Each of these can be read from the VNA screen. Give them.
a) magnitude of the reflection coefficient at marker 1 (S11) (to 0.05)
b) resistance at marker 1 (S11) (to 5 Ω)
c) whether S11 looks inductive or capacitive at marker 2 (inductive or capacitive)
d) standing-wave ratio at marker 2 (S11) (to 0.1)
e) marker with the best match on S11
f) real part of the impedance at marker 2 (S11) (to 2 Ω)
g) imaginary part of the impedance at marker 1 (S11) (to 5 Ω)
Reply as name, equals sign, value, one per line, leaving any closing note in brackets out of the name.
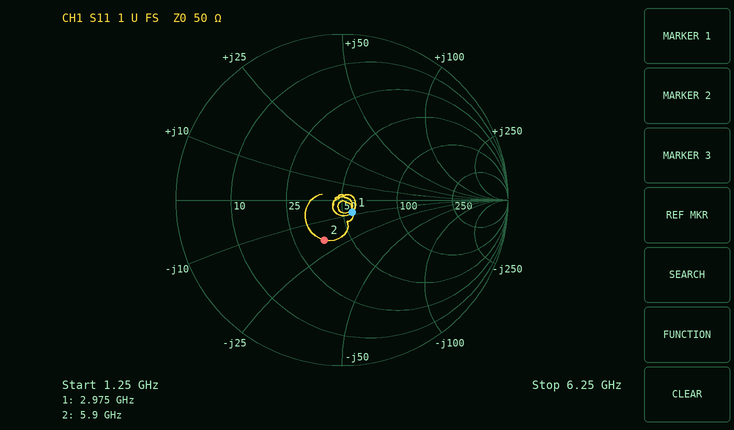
magnitude of the reflection coefficient at marker 1 (S11) = 0.10
resistance at marker 1 (S11) = 55 Ω
whether S11 looks inductive or capacitive at marker 2 = capacitive
standing-wave ratio at marker 2 (S11) = 1.7
marker with the best match on S11 = marker 1
real part of the impedance at marker 2 (S11) = 36 Ω
imaginary part of the impedance at marker 1 (S11) = -10 Ω
